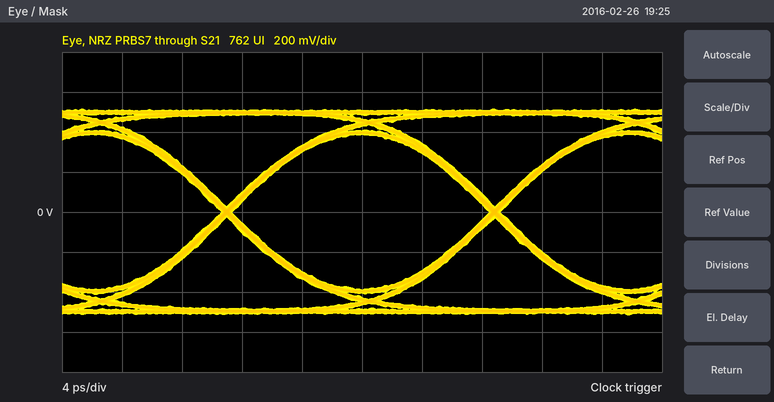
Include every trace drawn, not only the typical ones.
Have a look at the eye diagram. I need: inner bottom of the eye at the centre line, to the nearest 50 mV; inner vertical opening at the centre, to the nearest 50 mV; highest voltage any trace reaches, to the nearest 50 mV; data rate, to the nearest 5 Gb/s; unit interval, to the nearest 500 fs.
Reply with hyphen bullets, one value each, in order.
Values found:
- -400 mV
- 800 mV
- 500 mV
- 55 Gb/s
- 18.0 ps
